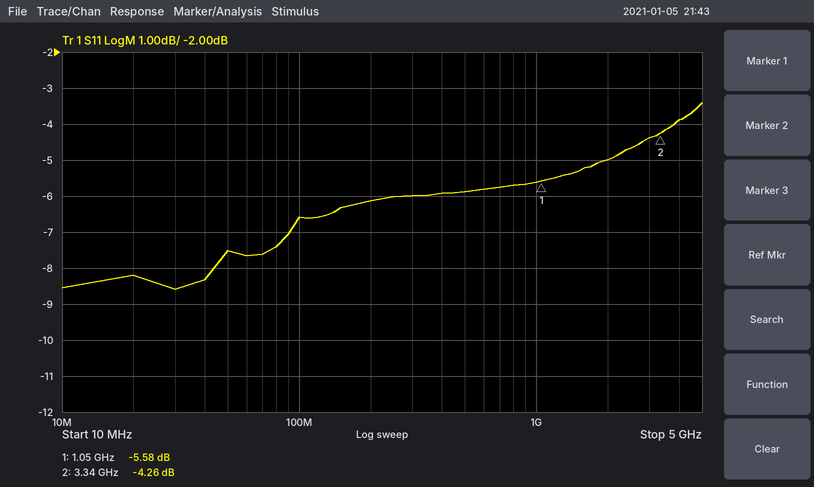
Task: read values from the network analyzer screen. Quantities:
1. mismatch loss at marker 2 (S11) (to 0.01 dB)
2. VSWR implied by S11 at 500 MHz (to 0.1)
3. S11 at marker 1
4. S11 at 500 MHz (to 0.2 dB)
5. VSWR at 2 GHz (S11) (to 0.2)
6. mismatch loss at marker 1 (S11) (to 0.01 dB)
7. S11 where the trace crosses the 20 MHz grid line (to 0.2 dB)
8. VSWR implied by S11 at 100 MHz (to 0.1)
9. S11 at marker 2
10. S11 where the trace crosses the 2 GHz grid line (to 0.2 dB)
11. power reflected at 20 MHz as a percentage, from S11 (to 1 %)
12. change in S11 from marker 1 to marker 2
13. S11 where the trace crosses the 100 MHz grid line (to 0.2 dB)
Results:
2.04 dB
3.1
-5.58 dB
-5.8 dB
3.6
1.41 dB
-8.2 dB
2.8
-4.26 dB
-5.0 dB
15 %
1.32 dB
-6.6 dB
